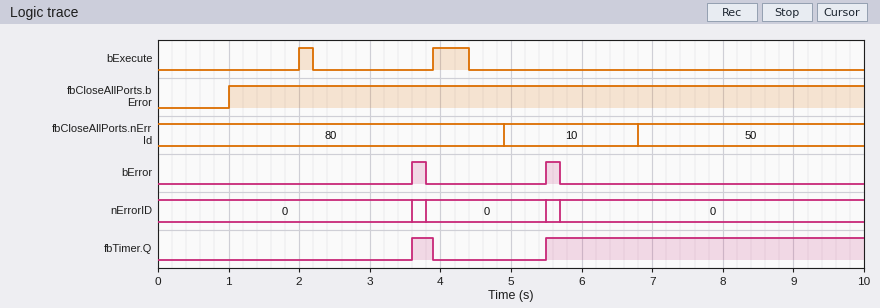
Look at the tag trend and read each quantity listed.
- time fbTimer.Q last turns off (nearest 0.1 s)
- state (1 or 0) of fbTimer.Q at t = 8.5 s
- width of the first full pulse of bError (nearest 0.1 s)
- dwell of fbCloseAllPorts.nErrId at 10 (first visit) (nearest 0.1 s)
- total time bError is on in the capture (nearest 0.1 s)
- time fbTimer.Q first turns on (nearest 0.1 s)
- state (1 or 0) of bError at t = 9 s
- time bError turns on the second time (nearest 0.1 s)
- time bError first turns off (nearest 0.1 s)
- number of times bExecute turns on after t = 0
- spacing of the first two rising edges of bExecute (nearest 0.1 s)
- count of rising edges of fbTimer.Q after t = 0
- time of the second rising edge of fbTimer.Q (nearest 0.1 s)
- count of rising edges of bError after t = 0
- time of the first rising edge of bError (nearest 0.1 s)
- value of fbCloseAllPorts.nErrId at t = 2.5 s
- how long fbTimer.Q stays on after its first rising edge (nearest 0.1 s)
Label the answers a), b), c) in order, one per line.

a) 3.9 s
b) 1
c) 0.2 s
d) 1.9 s
e) 0.4 s
f) 3.6 s
g) 0
h) 5.5 s
i) 3.8 s
j) 2
k) 1.9 s
l) 2
m) 5.5 s
n) 2
o) 3.6 s
p) 80
q) 0.3 s
